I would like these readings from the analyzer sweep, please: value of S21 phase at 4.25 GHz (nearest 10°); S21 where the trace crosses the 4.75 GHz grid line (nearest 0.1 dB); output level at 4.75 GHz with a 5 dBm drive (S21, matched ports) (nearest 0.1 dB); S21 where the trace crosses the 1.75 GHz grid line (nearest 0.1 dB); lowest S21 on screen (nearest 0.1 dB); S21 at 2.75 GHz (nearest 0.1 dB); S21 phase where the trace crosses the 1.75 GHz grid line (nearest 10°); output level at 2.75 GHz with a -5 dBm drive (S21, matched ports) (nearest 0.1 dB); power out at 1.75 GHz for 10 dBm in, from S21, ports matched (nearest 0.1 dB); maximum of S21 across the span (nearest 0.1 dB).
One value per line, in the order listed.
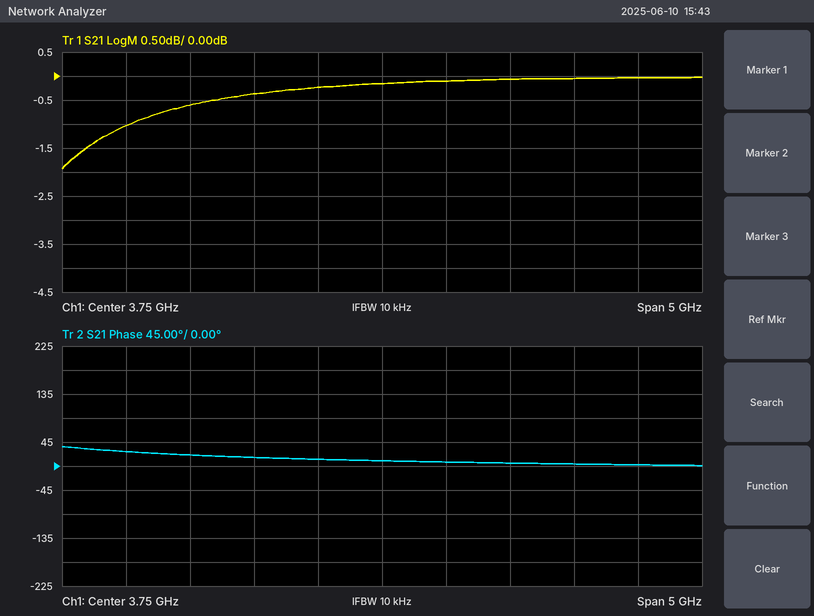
10°
-0.1 dB
4.9 dBm
-1.0 dB
-1.9 dB
-0.4 dB
30°
-5.4 dBm
9.0 dBm
0.0 dB
